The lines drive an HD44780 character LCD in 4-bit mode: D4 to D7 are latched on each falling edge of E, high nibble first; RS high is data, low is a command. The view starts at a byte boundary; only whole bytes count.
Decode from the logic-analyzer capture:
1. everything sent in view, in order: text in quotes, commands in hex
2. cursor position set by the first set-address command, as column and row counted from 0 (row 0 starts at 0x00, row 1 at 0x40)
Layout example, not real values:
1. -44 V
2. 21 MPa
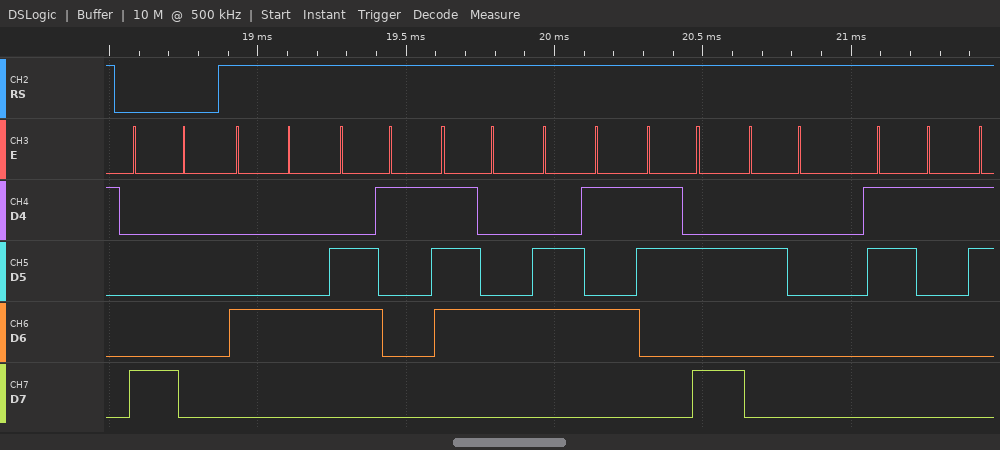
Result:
1. 0x80 "Date: 1"
2. column 0, row 0
